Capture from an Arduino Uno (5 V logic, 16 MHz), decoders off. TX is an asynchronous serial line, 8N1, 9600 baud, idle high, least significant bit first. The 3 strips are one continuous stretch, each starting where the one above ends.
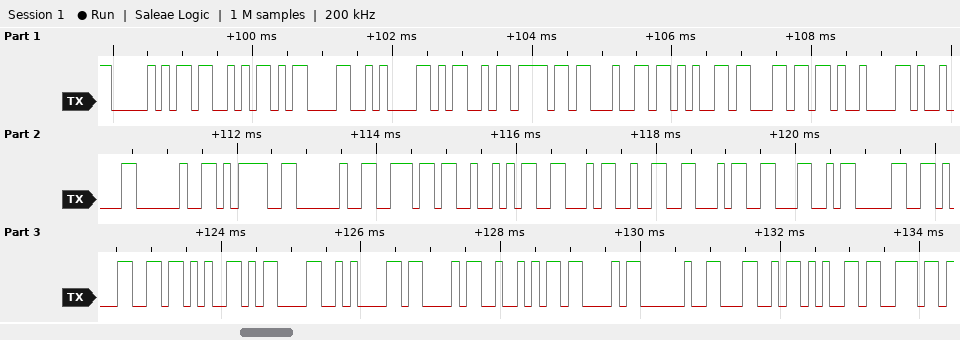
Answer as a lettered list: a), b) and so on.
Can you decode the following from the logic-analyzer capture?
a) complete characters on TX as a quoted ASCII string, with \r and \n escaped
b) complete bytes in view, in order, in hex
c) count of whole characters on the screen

a) "PS\r\nModel\t\t = nRF24L01+\r\nCRC Len"
b) 50 53 0D 0A 4D 6F 64 65 6C 09 09 20 3D 20 6E 52 46 32 34 4C 30 31 2B 0D 0A 43 52 43 20 4C 65 6E
c) 32
